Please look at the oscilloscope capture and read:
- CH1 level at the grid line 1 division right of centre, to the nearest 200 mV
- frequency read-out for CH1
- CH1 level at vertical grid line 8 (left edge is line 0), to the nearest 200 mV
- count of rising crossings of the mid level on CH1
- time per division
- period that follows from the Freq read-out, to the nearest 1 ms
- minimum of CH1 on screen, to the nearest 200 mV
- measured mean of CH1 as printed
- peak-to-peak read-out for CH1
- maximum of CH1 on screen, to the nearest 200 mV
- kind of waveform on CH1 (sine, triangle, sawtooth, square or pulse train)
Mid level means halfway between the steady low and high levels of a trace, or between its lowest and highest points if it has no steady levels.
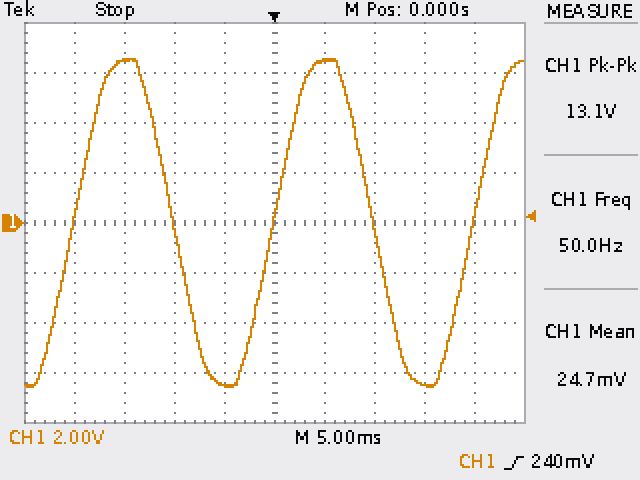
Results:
6.4 V
50.0 Hz
-6.4 V
3
5 ms
20 ms
-6.6 V
24.7 mV
13.1 V
6.6 V
sine
